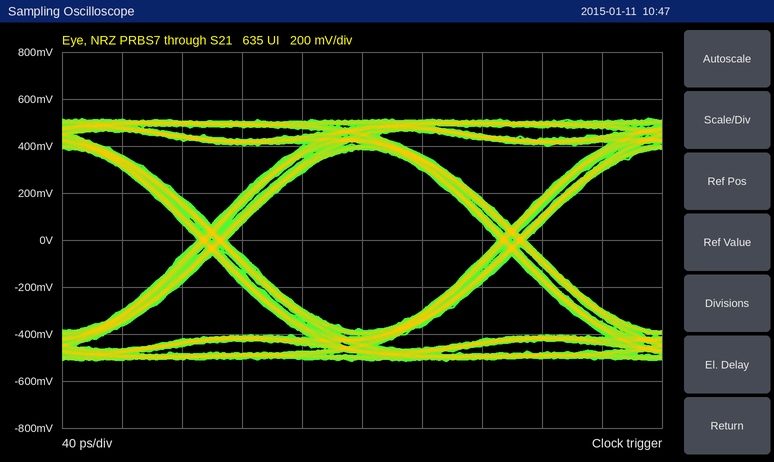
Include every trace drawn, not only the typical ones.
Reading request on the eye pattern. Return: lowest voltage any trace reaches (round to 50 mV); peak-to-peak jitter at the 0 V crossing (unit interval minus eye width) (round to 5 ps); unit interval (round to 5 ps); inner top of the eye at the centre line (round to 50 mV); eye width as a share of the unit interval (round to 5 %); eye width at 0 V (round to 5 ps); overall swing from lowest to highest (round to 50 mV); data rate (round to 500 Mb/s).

-500 mV
20 ps
200 ps
400 mV
90 %
180 ps
1.05 V
5.0 Gb/s
